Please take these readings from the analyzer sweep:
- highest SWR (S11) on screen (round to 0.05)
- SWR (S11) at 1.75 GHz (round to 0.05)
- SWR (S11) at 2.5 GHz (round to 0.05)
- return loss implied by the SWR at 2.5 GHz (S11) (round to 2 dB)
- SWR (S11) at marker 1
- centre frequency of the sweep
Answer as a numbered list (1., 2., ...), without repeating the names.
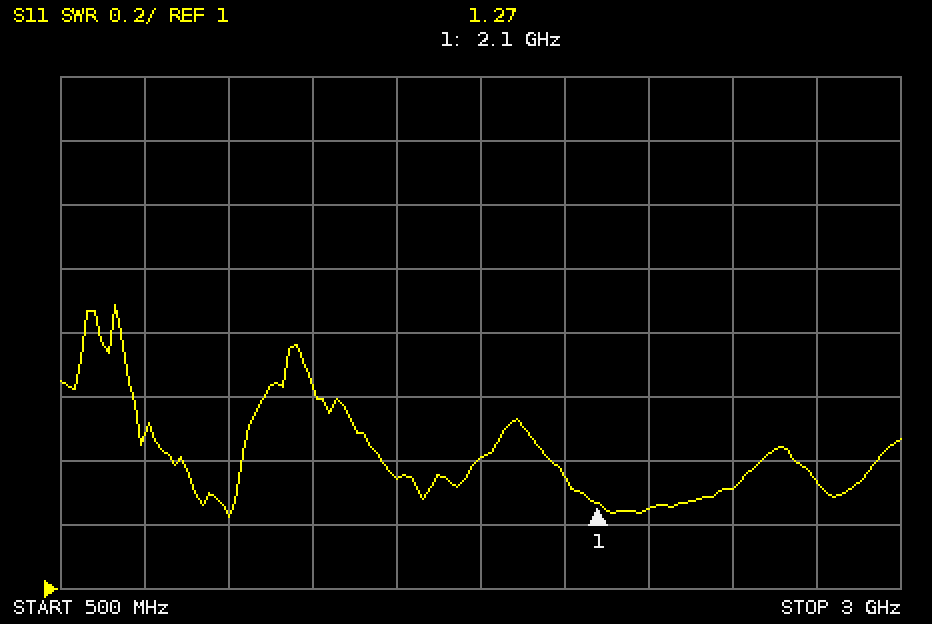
1. 1.90
2. 1.40
3. 1.30
4. 18 dB
5. 1.27
6. 1.75 GHz
